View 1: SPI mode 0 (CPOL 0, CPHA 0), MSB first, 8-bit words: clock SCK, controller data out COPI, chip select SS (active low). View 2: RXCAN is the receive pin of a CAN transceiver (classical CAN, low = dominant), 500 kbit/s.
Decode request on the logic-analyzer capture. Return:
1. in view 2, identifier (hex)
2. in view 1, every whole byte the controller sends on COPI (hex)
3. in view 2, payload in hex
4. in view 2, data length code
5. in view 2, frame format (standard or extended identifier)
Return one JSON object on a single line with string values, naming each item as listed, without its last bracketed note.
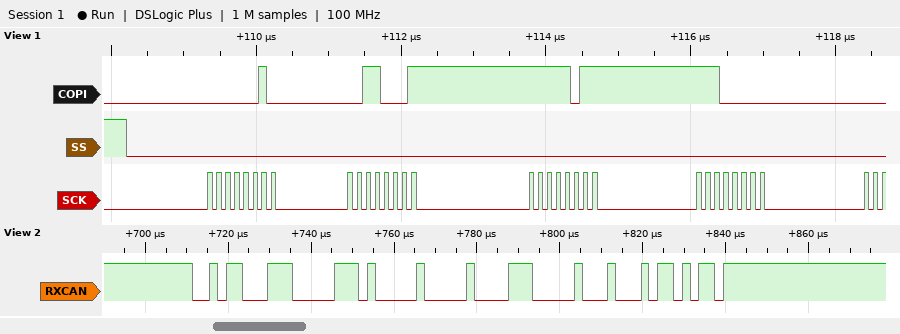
{"in view 2, identifier": "0x2C7", "in view 1, every whole byte the controller sends on COPI": "0x02 0x31 0xFB 0xE0", "in view 2, payload in hex": "40 00 E0", "in view 2, data length code": "3", "in view 2, frame format": "standard"}
